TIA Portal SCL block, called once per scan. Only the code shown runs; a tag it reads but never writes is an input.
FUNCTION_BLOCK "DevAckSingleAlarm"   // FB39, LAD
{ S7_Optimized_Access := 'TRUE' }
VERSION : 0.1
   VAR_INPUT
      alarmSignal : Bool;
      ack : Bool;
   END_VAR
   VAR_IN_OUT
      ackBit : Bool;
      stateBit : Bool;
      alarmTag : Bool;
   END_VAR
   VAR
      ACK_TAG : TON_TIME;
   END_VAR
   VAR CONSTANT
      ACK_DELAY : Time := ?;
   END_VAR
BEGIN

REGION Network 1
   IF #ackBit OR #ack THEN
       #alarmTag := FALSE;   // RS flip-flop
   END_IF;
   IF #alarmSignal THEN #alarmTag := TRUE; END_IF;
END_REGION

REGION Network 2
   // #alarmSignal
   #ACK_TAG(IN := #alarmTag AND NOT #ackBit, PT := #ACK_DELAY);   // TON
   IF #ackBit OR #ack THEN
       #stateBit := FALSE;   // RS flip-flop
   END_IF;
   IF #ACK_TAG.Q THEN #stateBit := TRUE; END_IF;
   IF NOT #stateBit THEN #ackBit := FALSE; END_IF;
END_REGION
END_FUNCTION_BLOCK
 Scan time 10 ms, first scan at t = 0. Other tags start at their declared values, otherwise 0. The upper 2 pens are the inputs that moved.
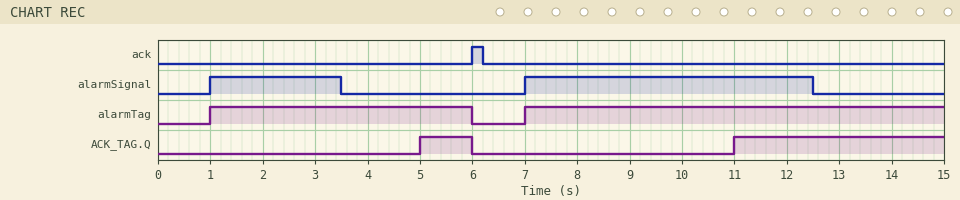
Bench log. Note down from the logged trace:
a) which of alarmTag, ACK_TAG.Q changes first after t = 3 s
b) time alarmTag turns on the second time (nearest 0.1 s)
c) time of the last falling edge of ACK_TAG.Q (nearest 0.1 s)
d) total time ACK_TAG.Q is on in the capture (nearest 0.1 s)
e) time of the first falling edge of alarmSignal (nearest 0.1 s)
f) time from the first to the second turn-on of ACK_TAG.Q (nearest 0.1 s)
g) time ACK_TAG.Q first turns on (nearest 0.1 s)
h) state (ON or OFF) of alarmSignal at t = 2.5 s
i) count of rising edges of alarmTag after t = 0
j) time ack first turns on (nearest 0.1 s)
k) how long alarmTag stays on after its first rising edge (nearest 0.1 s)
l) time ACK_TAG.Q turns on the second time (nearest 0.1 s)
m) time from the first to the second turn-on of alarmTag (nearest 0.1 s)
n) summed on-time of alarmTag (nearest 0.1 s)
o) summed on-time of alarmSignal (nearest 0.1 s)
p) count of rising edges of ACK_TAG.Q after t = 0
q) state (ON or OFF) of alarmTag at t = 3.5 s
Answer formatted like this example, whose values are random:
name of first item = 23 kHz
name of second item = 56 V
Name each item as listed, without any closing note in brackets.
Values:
which of alarmTag, ACK_TAG.Q changes first after t = 3 s = ACK_TAG.Q
time alarmTag turns on the second time = 7.0 s
time of the last falling edge of ACK_TAG.Q = 6.0 s
total time ACK_TAG.Q is on in the capture = 5.0 s
time of the first falling edge of alarmSignal = 3.5 s
time from the first to the second turn-on of ACK_TAG.Q = 6.0 s
time ACK_TAG.Q first turns on = 5.0 s
state (ON or OFF) of alarmSignal at t = 2.5 s = ON
count of rising edges of alarmTag after t = 0 = 2
time ack first turns on = 6.0 s
how long alarmTag stays on after its first rising edge = 5.0 s
time ACK_TAG.Q turns on the second time = 11.0 s
time from the first to the second turn-on of alarmTag = 6.0 s
summed on-time of alarmTag = 13.0 s
summed on-time of alarmSignal = 8.0 s
count of rising edges of ACK_TAG.Q after t = 0 = 2
state (ON or OFF) of alarmTag at t = 3.5 s = ON
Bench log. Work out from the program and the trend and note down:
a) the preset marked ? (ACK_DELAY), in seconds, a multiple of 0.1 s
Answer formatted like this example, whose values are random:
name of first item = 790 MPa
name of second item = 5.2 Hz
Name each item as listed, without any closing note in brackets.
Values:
the preset marked ? (ACK_DELAY), in seconds, a multiple of 0.1 s = 4.0 s
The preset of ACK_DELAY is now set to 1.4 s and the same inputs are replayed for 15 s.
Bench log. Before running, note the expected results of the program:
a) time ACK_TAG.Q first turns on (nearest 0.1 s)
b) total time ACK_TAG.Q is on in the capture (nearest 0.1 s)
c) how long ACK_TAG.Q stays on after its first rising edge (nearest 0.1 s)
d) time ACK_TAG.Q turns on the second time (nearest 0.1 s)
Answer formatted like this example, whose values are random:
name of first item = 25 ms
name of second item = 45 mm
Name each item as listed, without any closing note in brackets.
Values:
time ACK_TAG.Q first turns on = 2.4 s
total time ACK_TAG.Q is on in the capture = 10.2 s
how long ACK_TAG.Q stays on after its first rising edge = 3.6 s
time ACK_TAG.Q turns on the second time = 8.4 s
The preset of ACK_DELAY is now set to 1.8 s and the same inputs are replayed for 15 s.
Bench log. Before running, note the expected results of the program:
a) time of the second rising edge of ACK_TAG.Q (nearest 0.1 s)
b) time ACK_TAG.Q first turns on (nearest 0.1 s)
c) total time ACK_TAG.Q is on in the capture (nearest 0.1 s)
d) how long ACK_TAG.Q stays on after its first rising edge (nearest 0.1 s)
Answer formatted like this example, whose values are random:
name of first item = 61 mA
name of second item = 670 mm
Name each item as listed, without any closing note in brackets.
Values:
time of the second rising edge of ACK_TAG.Q = 8.8 s
time ACK_TAG.Q first turns on = 2.8 s
total time ACK_TAG.Q is on in the capture = 9.4 s
how long ACK_TAG.Q stays on after its first rising edge = 3.2 s
